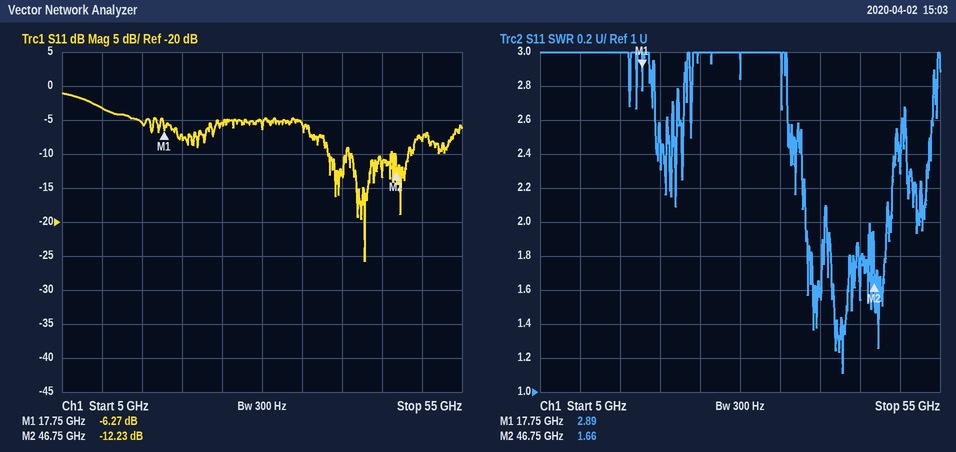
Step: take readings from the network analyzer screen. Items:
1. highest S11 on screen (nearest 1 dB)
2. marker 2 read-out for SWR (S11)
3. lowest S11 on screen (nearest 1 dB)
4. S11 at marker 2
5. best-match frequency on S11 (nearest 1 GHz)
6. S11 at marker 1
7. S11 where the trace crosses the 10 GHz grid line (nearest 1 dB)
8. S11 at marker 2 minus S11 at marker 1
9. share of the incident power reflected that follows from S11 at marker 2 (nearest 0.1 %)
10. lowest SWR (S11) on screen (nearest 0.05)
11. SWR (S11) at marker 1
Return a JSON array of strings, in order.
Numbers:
["-1 dB", "1.66", "-26 dB", "-12.23 dB", "43 GHz", "-6.27 dB", "-3 dB", "-5.96 dB", "6.0 %", "1.10", "2.89"]
